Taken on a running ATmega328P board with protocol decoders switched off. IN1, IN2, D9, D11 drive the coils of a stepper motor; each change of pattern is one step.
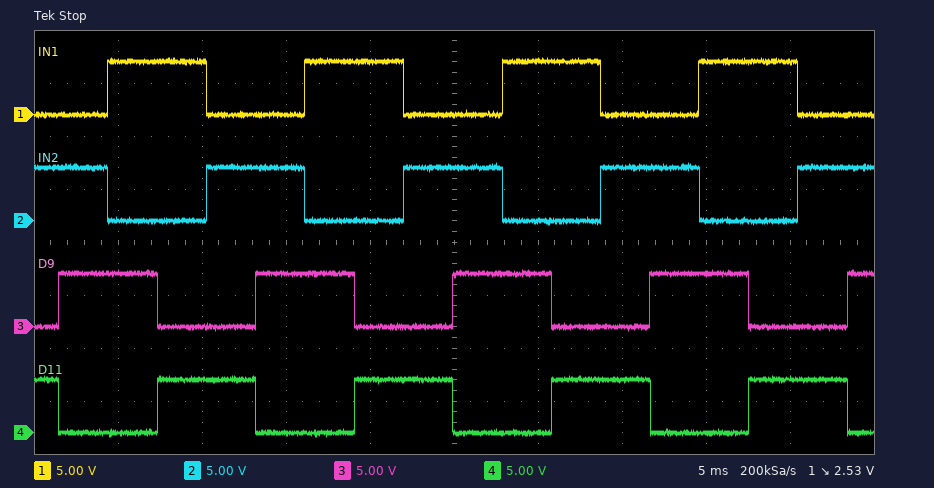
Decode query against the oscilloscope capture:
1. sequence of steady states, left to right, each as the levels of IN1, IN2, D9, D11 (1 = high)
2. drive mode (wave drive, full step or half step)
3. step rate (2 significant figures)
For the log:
0101 0110 1010 1001 0101 0110 1010 1001 0101 0110 1010 1001 0101 0110 1010 1001 0101 0110
full step
340 steps/s
